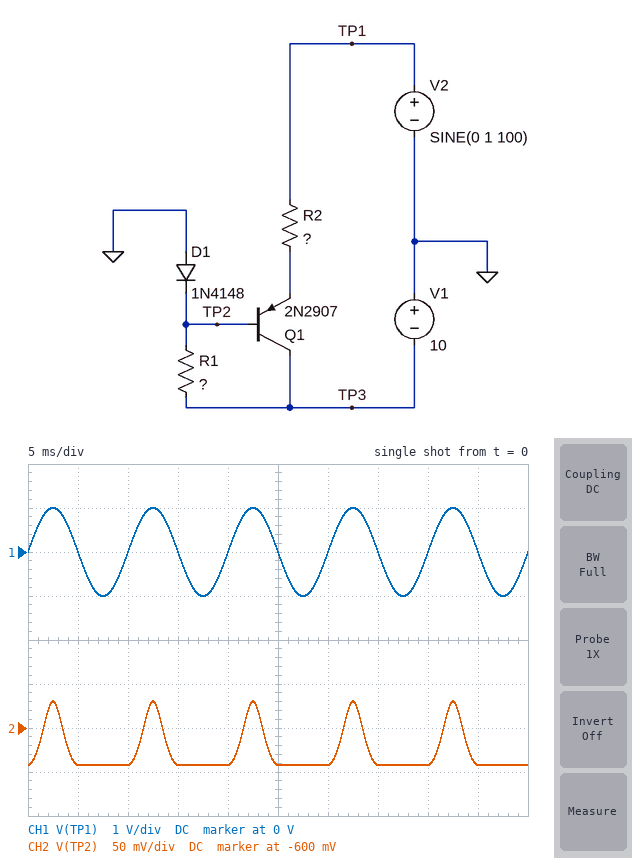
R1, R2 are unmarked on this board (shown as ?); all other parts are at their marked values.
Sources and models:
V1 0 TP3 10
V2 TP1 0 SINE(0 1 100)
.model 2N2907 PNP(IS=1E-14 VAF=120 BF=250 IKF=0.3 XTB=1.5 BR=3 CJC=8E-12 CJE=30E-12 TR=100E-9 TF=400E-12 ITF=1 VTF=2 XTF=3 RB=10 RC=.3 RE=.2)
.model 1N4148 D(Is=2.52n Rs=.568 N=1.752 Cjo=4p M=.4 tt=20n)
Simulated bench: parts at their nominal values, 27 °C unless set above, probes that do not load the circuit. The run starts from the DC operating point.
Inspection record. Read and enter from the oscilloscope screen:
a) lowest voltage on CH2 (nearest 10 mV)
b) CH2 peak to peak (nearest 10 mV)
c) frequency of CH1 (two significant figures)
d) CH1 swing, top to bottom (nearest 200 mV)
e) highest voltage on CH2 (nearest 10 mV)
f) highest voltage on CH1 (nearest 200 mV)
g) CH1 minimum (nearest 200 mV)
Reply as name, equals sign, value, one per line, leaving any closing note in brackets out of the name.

lowest voltage on CH2 = -640 mV
CH2 peak to peak = 70 mV
frequency of CH1 = 100 Hz
CH1 swing, top to bottom = 2.0 V
highest voltage on CH2 = -570 mV
highest voltage on CH1 = 1.0 V
CH1 minimum = -1.0 V
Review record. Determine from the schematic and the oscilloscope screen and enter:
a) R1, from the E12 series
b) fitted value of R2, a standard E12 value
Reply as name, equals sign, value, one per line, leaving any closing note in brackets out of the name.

R1, from the E12 series = 2.7 kΩ
fitted value of R2, a standard E12 value = 1.8 Ω
